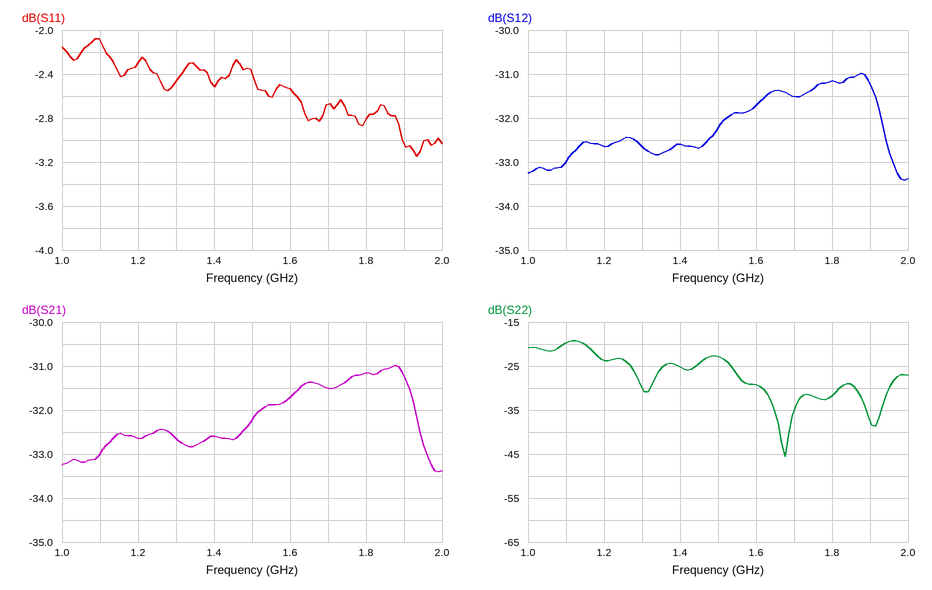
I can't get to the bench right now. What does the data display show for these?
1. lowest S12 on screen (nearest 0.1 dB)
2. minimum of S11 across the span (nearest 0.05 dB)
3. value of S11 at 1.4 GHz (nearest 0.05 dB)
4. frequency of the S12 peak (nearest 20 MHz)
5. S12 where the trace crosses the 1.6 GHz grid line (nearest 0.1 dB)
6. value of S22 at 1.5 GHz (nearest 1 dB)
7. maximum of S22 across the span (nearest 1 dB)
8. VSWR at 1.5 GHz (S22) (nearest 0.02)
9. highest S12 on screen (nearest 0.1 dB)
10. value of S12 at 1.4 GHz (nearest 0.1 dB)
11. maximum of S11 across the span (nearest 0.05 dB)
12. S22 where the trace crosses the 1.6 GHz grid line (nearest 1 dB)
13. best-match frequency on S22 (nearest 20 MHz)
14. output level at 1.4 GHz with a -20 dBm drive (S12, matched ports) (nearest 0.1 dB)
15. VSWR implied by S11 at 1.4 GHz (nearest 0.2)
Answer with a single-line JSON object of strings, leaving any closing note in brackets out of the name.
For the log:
{"lowest S12 on screen": "-33.4 dB", "minimum of S11 across the span": "-3.15 dB", "value of S11 at 1.4 GHz": "-2.50 dB", "frequency of the S12 peak": "1.88 GHz", "S12 where the trace crosses the 1.6 GHz grid line": "-31.7 dB", "value of S22 at 1.5 GHz": "-23 dB", "maximum of S22 across the span": "-19 dB", "VSWR at 1.5 GHz (S22)": "1.16", "highest S12 on screen": "-31.0 dB", "value of S12 at 1.4 GHz": "-32.6 dB", "maximum of S11 across the span": "-2.10 dB", "S22 where the trace crosses the 1.6 GHz grid line": "-29 dB", "best-match frequency on S22": "1.68 GHz", "output level at 1.4 GHz with a -20 dBm drive (S12, matched ports)": "-52.6 dBm", "VSWR implied by S11 at 1.4 GHz": "7.0"}
